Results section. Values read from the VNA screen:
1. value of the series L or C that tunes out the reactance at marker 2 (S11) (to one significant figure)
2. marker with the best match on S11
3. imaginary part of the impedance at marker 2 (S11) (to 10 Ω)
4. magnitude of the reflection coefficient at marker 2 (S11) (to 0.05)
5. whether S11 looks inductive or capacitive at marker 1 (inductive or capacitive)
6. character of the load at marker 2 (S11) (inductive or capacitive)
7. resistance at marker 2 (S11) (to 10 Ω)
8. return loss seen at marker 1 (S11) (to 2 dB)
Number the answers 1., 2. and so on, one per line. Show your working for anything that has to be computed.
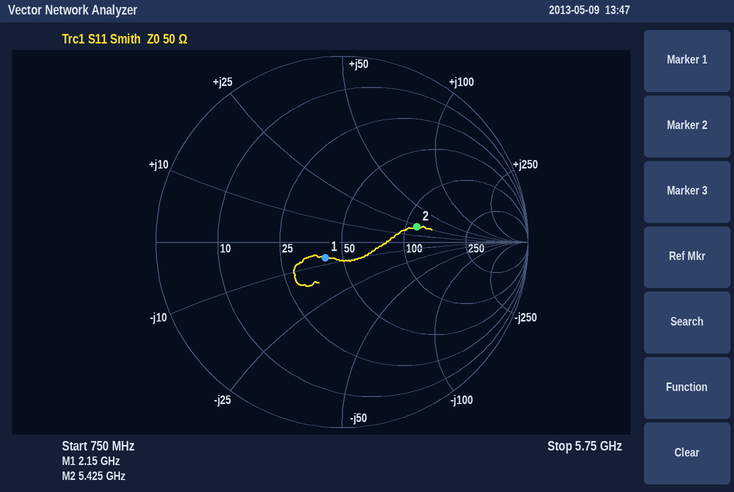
1. C = 1/(2π × 5.425 GHz × 20 Ω) ≈ 1 pF
2. marker 1
3. +20 Ω
4. 0.40
5. capacitive
6. inductive
7. 110 Ω
8. 18 dB
